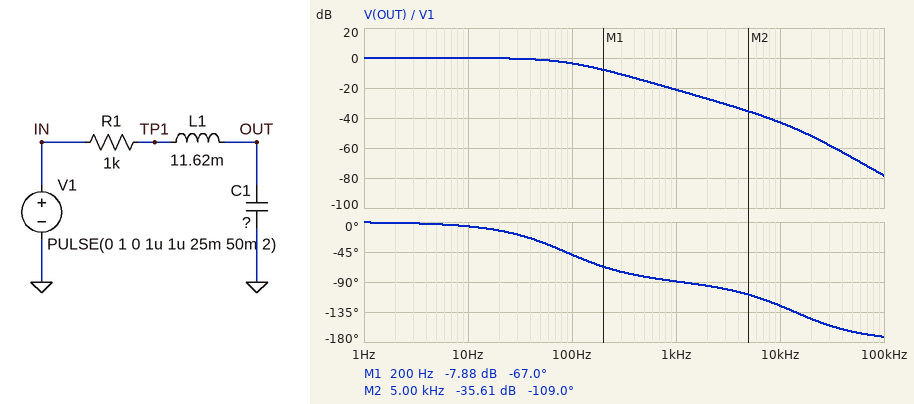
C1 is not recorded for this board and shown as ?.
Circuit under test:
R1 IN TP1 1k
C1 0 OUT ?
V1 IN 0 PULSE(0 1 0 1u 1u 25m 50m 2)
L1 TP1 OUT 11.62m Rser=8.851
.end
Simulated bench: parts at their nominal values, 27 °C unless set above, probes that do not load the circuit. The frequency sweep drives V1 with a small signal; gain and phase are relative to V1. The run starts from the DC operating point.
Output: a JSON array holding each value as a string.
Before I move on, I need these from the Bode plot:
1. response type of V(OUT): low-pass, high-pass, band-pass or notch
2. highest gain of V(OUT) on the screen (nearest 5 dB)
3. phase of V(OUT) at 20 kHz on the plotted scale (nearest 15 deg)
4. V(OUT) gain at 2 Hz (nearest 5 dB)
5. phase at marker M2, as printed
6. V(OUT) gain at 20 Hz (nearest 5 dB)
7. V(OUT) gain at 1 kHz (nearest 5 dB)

["low-pass", "0 dB", "-150 deg", "0 dB", "-109.0 deg", "0 dB", "-20 dB"]
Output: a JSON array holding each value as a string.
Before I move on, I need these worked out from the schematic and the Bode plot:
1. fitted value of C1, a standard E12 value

["1.8 µF"]
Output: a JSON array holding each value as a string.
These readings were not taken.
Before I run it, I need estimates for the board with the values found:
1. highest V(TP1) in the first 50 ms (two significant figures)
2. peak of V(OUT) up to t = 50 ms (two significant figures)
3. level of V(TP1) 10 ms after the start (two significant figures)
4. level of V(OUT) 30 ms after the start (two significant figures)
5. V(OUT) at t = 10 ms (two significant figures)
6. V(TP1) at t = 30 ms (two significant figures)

["1.0 V", "1.0 V", "1.0 V", "63 mV", "1.0 V", "63 mV"]
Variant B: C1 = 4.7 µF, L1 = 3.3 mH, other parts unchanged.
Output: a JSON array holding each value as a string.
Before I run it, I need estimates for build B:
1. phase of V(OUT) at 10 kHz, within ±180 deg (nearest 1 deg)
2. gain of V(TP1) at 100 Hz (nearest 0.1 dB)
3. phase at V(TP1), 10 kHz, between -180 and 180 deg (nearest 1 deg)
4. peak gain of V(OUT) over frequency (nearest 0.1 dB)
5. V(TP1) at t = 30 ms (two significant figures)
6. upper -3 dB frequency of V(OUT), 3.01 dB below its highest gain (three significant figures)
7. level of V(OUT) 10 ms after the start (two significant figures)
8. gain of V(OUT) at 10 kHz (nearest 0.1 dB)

["-101 deg", "-10.0 dB", "76 deg", "0 dB", "340 mV", "33.6 Hz", "880 mV", "-49.7 dB"]
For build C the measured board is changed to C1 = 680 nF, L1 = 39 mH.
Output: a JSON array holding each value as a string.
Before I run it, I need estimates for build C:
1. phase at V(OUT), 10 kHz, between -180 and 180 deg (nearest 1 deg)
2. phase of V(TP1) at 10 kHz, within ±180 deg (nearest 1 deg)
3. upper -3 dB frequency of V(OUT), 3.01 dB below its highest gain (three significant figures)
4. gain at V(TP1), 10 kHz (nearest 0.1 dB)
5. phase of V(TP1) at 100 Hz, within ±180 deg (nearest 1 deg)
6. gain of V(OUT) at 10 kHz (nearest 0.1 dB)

["-157 deg", "22 deg", "246 Hz", "-0.7 dB", "-23 deg", "-41.0 dB"]
